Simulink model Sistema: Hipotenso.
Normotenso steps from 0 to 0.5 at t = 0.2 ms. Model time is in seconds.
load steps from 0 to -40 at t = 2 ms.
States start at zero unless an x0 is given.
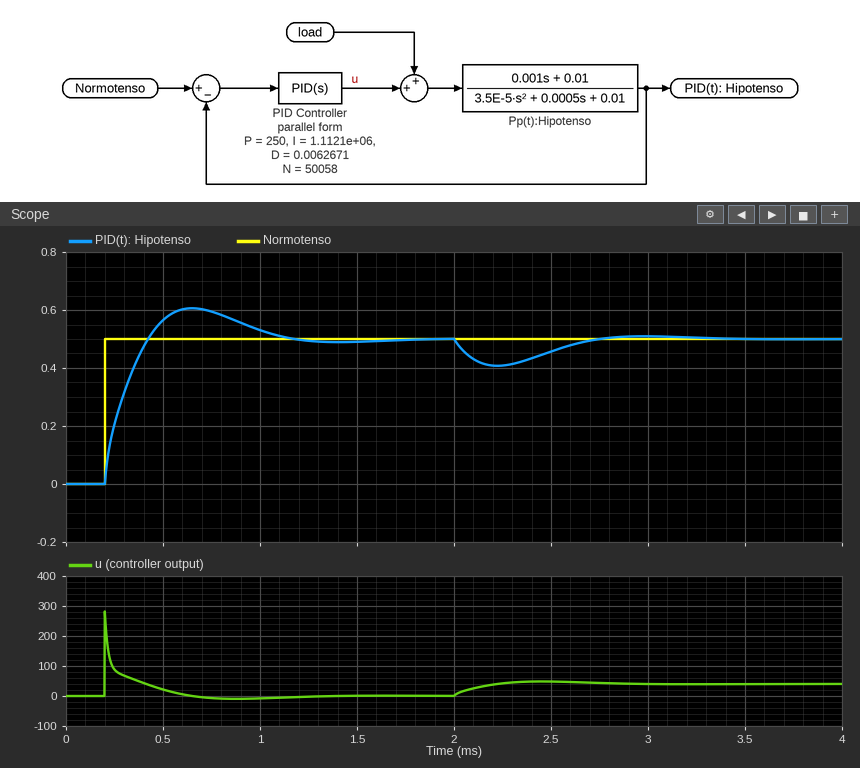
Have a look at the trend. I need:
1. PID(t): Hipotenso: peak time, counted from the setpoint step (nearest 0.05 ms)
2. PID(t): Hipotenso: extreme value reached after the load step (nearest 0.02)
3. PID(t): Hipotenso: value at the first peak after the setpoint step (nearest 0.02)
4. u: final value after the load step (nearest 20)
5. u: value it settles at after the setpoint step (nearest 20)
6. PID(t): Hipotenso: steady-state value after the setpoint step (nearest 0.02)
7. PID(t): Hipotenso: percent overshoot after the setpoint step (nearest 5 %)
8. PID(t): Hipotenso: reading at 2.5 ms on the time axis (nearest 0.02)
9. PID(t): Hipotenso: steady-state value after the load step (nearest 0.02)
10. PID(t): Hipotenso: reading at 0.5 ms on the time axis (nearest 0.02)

0.45 ms
0.40
0.60
40
0
0.50
20 %
0.46
0.50
0.56
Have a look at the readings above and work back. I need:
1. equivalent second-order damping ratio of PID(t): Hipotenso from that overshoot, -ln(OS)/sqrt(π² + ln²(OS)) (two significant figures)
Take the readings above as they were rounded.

0.46
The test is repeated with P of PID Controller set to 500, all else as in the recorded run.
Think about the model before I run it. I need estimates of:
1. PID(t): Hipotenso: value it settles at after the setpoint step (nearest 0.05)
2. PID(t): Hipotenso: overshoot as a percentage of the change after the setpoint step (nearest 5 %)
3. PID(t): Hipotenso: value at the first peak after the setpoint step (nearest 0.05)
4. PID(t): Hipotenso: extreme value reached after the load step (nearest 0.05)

0.50
10 %
0.55
0.45
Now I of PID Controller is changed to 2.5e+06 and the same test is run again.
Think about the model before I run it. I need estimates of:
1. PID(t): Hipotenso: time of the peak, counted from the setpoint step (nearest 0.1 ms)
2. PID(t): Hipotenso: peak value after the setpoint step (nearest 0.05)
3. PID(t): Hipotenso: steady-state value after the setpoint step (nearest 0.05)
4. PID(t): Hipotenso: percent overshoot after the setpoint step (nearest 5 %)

0.3 ms
0.65
0.50
30 %
